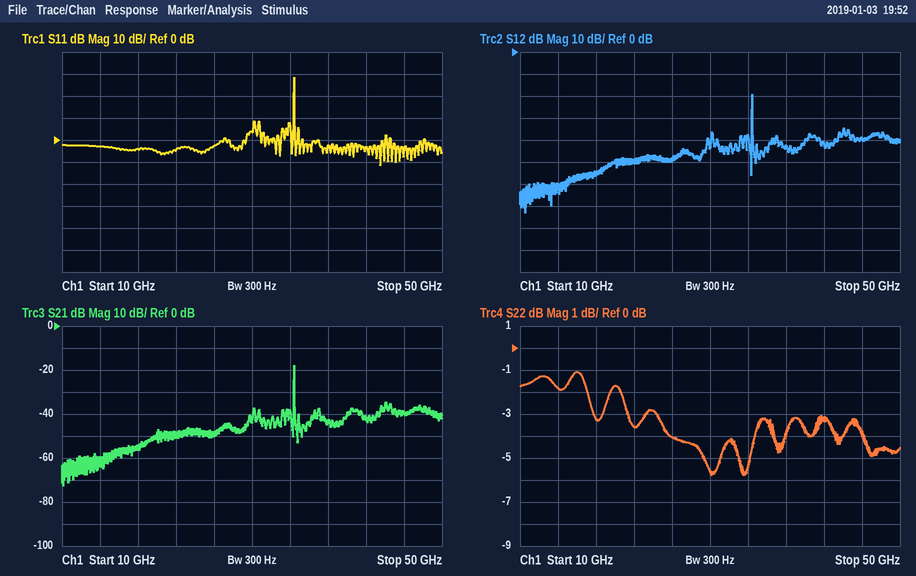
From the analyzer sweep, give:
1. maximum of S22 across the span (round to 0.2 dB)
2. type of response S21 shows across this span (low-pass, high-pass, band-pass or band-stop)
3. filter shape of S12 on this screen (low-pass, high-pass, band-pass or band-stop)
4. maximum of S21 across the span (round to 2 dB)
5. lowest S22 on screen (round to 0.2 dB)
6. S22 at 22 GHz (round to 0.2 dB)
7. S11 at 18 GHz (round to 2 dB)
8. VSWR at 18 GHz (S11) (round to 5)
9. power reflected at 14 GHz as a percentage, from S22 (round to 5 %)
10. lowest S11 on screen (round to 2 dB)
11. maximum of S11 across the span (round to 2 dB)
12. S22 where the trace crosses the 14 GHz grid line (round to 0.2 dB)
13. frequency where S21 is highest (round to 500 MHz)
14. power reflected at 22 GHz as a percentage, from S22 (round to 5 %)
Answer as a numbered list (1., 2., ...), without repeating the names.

1. -1.0 dB
2. band-pass
3. band-pass
4. -18 dB
5. -5.8 dB
6. -3.6 dB
7. -4 dB
8. 5
9. 65 %
10. -12 dB
11. 28 dB
12. -1.8 dB
13. 34.5 GHz
14. 45 %
